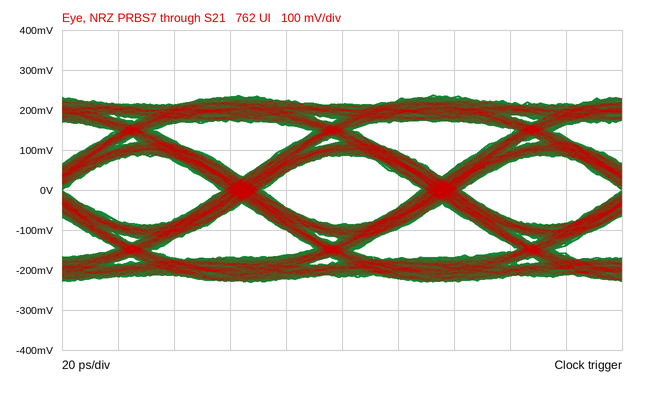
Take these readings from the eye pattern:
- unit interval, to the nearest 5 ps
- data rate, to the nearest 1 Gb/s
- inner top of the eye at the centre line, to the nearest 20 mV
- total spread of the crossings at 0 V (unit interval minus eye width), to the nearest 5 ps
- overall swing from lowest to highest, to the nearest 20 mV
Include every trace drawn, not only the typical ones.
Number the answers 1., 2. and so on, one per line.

1. 70 ps
2. 14 Gb/s
3. 80 mV
4. 15 ps
5. 460 mV
